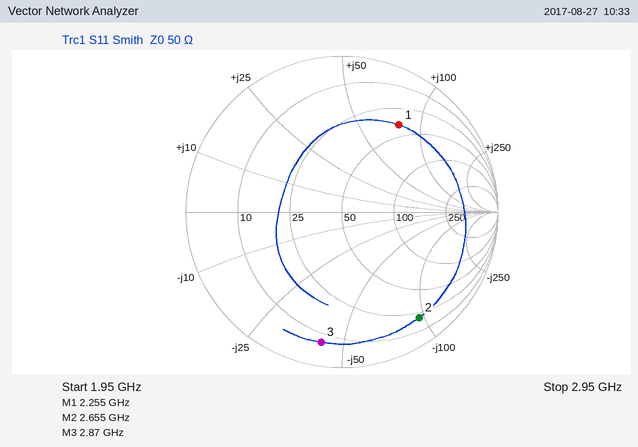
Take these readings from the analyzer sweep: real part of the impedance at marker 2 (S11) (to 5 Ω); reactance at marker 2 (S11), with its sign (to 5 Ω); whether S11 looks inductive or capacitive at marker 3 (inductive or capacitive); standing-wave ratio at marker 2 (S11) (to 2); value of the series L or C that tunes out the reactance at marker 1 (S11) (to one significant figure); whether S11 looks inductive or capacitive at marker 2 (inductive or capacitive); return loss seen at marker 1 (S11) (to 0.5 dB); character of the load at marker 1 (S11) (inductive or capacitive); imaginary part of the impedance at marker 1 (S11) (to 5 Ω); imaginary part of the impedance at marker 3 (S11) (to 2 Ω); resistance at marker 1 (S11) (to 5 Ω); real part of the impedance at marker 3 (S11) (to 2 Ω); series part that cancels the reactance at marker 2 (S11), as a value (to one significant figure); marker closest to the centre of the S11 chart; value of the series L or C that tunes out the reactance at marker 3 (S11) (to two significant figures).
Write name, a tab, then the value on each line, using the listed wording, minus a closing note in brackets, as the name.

real part of the impedance at marker 2 (S11)	20 Ω
reactance at marker 2 (S11), with its sign	-95 Ω
whether S11 looks inductive or capacitive at marker 3	capacitive
standing-wave ratio at marker 2 (S11)	12
value of the series L or C that tunes out the reactance at marker 1 (S11)	900 fF
whether S11 looks inductive or capacitive at marker 2	capacitive
return loss seen at marker 1 (S11)	3.5 dB
character of the load at marker 1 (S11)	inductive
imaginary part of the impedance at marker 1 (S11)	+80 Ω
imaginary part of the impedance at marker 3 (S11)	-42 Ω
resistance at marker 1 (S11)	40 Ω
real part of the impedance at marker 3 (S11)	8 Ω
series part that cancels the reactance at marker 2 (S11), as a value	6 nH
marker closest to the centre of the S11 chart	marker 1
value of the series L or C that tunes out the reactance at marker 3 (S11)	2.3 nH
